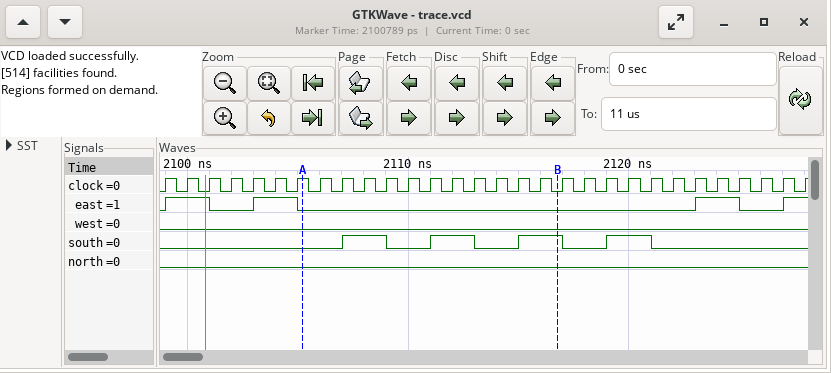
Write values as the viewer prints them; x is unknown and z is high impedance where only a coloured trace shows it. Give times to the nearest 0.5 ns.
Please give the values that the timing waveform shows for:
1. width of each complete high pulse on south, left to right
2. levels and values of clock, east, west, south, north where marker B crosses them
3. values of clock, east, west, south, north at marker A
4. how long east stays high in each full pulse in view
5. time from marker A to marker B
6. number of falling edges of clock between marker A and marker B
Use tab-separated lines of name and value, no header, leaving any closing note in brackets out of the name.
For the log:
width of each complete high pulse on south, left to right	2 ns, 2 ns, 2 ns, 2 ns
levels and values of clock, east, west, south, north where marker B crosses them	clock=0, east=0, west=0, south=1, north=0
values of clock, east, west, south, north at marker A	clock=1, east=0, west=0, south=0, north=0
how long east stays high in each full pulse in view	2 ns, 2 ns, 2 ns
time from marker A to marker B	11.5 ns
number of falling edges of clock between marker A and marker B	12
